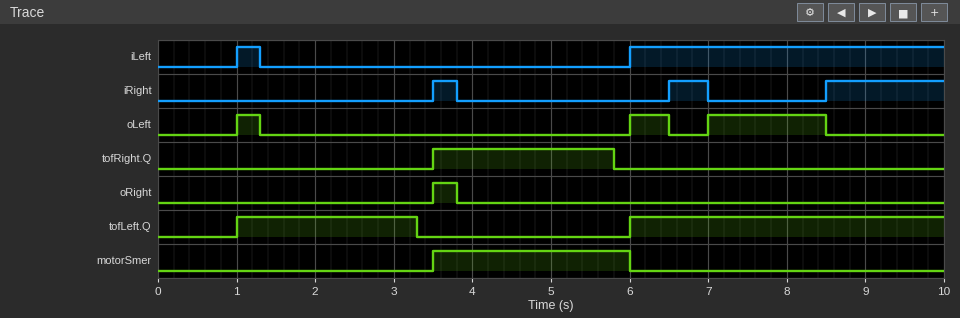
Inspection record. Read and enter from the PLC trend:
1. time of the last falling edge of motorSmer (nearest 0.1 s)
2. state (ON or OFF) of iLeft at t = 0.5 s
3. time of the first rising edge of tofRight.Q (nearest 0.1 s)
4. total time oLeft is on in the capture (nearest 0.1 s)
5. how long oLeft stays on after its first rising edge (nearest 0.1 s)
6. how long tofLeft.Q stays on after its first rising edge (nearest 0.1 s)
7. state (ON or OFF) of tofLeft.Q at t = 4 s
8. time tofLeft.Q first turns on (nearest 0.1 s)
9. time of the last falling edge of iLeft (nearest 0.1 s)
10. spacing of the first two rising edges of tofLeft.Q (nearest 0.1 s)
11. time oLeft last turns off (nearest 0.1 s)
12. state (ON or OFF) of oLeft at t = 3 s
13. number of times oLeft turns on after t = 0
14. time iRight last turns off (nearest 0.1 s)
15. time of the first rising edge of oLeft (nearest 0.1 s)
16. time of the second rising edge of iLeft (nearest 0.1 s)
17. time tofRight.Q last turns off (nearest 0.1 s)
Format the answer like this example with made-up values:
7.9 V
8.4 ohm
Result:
6.0 s
OFF
3.5 s
2.3 s
0.3 s
2.3 s
OFF
1.0 s
1.3 s
5.0 s
8.5 s
OFF
3
7.0 s
1.0 s
6.0 s
5.8 s
